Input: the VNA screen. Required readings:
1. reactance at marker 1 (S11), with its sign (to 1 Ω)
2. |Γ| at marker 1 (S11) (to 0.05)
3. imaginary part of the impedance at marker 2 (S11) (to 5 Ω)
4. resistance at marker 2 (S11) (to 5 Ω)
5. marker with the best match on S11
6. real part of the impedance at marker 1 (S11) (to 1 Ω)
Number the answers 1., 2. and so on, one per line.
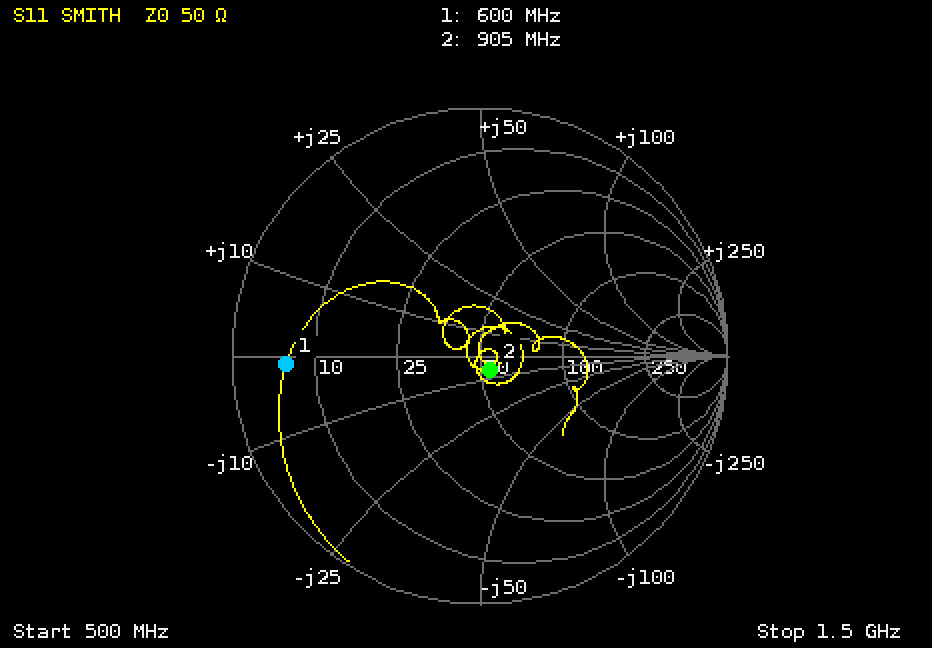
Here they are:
1. -1 Ω
2. 0.80
3. -5 Ω
4. 55 Ω
5. marker 2
6. 6 Ω
